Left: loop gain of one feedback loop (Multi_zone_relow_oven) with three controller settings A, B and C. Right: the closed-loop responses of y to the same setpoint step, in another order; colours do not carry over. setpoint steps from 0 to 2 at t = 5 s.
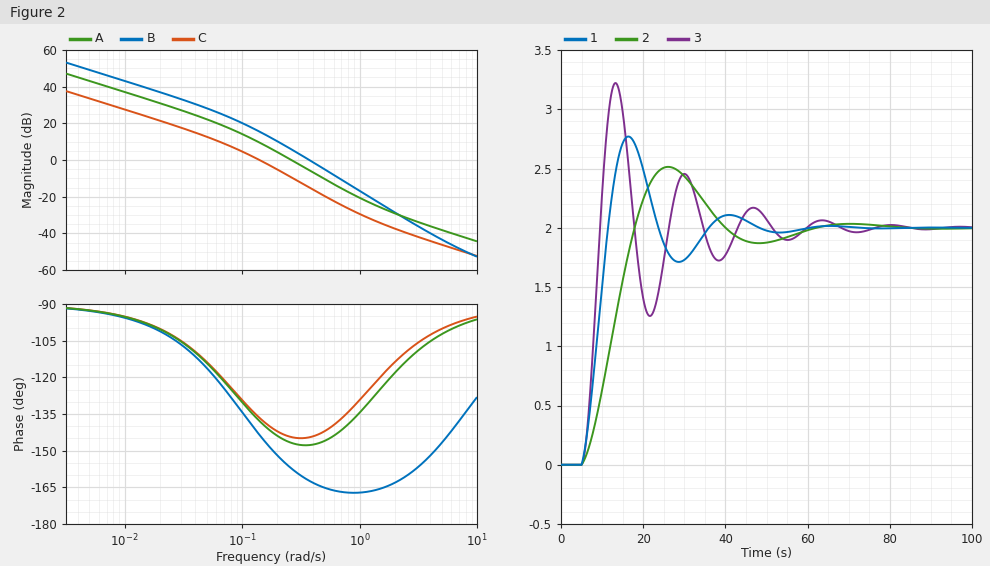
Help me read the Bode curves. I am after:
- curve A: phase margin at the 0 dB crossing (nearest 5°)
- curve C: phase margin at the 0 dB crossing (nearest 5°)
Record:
35°
45°
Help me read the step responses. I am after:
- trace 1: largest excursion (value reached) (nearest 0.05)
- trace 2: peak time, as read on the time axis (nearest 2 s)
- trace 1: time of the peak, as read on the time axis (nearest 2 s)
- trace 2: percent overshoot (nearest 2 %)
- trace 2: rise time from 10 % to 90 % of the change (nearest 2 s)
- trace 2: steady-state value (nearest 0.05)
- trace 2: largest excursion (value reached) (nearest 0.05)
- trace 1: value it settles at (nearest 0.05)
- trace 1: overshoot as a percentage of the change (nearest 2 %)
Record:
2.75
26 s
16 s
26 %
10 s
2.00
2.50
2.00
38 %
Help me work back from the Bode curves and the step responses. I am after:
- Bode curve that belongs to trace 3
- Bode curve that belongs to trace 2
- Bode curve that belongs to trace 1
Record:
B
C
A
